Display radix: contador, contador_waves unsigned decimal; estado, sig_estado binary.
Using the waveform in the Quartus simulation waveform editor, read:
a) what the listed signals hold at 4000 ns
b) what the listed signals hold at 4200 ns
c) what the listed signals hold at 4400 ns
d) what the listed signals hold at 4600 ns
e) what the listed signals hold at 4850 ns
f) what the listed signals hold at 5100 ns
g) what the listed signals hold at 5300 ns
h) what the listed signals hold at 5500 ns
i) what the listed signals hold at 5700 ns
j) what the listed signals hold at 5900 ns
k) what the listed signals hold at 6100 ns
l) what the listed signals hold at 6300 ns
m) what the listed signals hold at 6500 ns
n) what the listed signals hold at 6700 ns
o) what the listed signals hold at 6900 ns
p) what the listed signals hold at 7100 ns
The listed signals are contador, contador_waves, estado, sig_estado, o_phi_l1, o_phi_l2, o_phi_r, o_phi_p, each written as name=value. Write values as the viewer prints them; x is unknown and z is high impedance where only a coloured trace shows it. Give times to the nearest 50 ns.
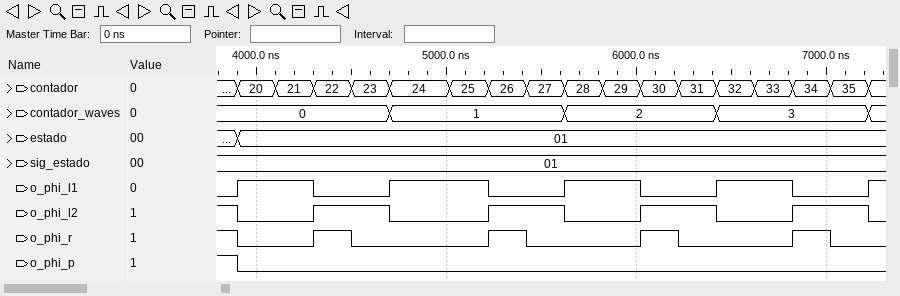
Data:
contador=20, contador_waves=0, estado=01, sig_estado=01, o_phi_l1=1, o_phi_l2=0, o_phi_r=0, o_phi_p=0
contador=21, contador_waves=0, estado=01, sig_estado=01, o_phi_l1=1, o_phi_l2=0, o_phi_r=0, o_phi_p=0
contador=22, contador_waves=0, estado=01, sig_estado=01, o_phi_l1=0, o_phi_l2=1, o_phi_r=1, o_phi_p=0
contador=23, contador_waves=0, estado=01, sig_estado=01, o_phi_l1=0, o_phi_l2=1, o_phi_r=0, o_phi_p=0
contador=24, contador_waves=1, estado=01, sig_estado=01, o_phi_l1=1, o_phi_l2=0, o_phi_r=0, o_phi_p=0
contador=25, contador_waves=1, estado=01, sig_estado=01, o_phi_l1=1, o_phi_l2=0, o_phi_r=0, o_phi_p=0
contador=26, contador_waves=1, estado=01, sig_estado=01, o_phi_l1=0, o_phi_l2=1, o_phi_r=1, o_phi_p=0
contador=27, contador_waves=1, estado=01, sig_estado=01, o_phi_l1=0, o_phi_l2=1, o_phi_r=0, o_phi_p=0
contador=28, contador_waves=2, estado=01, sig_estado=01, o_phi_l1=1, o_phi_l2=0, o_phi_r=0, o_phi_p=0
contador=29, contador_waves=2, estado=01, sig_estado=01, o_phi_l1=1, o_phi_l2=0, o_phi_r=0, o_phi_p=0
contador=30, contador_waves=2, estado=01, sig_estado=01, o_phi_l1=0, o_phi_l2=1, o_phi_r=1, o_phi_p=0
contador=31, contador_waves=2, estado=01, sig_estado=01, o_phi_l1=0, o_phi_l2=1, o_phi_r=0, o_phi_p=0
contador=32, contador_waves=3, estado=01, sig_estado=01, o_phi_l1=1, o_phi_l2=0, o_phi_r=0, o_phi_p=0
contador=33, contador_waves=3, estado=01, sig_estado=01, o_phi_l1=1, o_phi_l2=0, o_phi_r=0, o_phi_p=0
contador=34, contador_waves=3, estado=01, sig_estado=01, o_phi_l1=0, o_phi_l2=1, o_phi_r=1, o_phi_p=0
contador=35, contador_waves=3, estado=01, sig_estado=01, o_phi_l1=0, o_phi_l2=1, o_phi_r=0, o_phi_p=0
